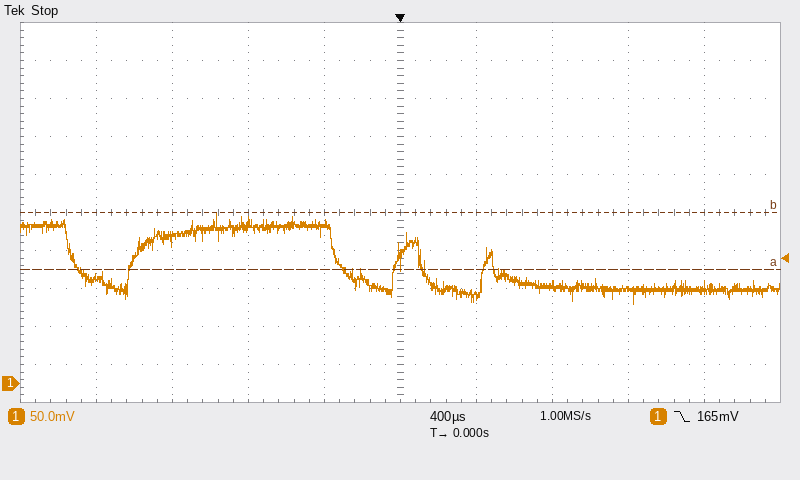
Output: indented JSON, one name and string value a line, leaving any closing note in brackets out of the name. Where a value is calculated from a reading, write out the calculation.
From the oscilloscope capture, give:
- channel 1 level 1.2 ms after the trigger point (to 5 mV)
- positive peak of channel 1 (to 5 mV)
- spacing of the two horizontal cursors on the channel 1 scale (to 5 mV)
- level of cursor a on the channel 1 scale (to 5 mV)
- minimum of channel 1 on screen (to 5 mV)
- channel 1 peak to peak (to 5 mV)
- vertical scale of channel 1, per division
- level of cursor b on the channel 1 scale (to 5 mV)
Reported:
{
  "channel 1 level 1.2 ms after the trigger point": "125 mV",
  "positive peak of channel 1": "225 mV",
  "spacing of the two horizontal cursors on the channel 1 scale": "75 mV",
  "level of cursor a on the channel 1 scale": "150 mV",
  "minimum of channel 1 on screen": "105 mV",
  "channel 1 peak to peak": "225 mV − (105 mV) = 120 mV",
  "vertical scale of channel 1, per division": "50 mV",
  "level of cursor b on the channel 1 scale": "225 mV"
}
